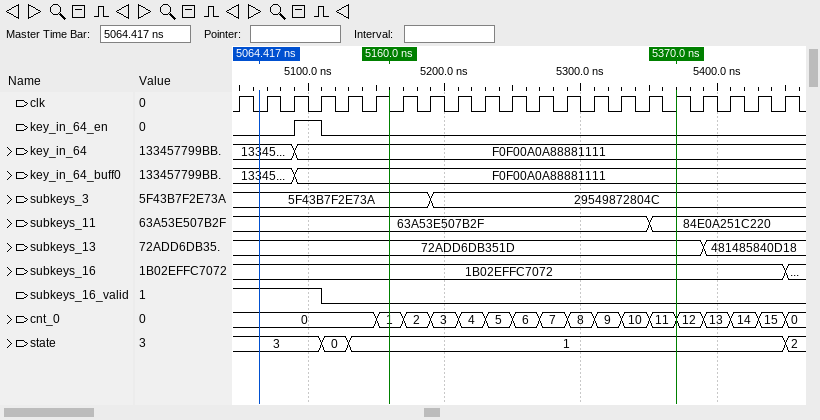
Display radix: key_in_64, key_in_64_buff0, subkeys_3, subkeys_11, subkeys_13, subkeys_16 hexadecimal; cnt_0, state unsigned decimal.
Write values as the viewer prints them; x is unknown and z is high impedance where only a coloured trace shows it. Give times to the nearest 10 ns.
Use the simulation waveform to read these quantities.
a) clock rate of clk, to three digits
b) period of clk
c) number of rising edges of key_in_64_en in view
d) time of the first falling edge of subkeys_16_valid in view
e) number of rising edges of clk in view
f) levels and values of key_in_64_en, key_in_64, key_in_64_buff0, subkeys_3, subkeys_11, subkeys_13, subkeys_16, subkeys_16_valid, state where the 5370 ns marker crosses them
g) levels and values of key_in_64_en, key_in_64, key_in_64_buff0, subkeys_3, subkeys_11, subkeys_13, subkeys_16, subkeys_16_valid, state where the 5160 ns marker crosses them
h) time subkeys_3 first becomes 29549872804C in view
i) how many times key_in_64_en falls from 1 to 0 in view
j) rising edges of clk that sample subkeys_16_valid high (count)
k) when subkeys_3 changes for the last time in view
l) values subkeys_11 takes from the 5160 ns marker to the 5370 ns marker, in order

50.0 MHz
20 ns
1
5110 ns
21
key_in_64_en=0, key_in_64=F0F00A0A88881111, key_in_64_buff0=F0F00A0A88881111, subkeys_3=29549872804C, subkeys_11=84E0A251C220, subkeys_13=72ADD6DB351D, subkeys_16=1B02EFFC7072, subkeys_16_valid=0, state=1
key_in_64_en=0, key_in_64=F0F00A0A88881111, key_in_64_buff0=F0F00A0A88881111, subkeys_3=5F43B7F2E73A, subkeys_11=63A53E507B2F, subkeys_13=72ADD6DB351D, subkeys_16=1B02EFFC7072, subkeys_16_valid=0, state=1
5190 ns
1
4
5190 ns
63A53E507B2F, 84E0A251C220
